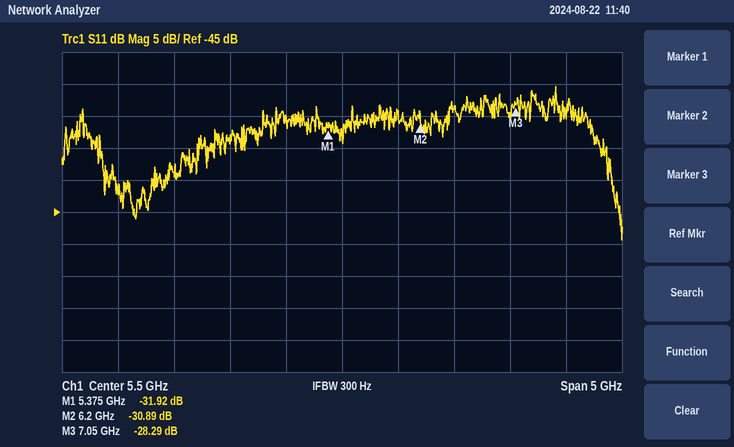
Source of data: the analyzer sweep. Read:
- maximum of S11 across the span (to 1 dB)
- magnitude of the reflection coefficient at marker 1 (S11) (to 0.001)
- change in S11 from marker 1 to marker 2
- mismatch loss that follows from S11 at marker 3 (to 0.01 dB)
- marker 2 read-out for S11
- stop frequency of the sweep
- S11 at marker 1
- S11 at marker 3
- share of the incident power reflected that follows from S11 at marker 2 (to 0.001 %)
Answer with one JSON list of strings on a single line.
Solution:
["-25 dB", "0.025", "1.03 dB", "0.01 dB", "-30.89 dB", "8 GHz", "-31.92 dB", "-28.29 dB", "0.081 %"]
